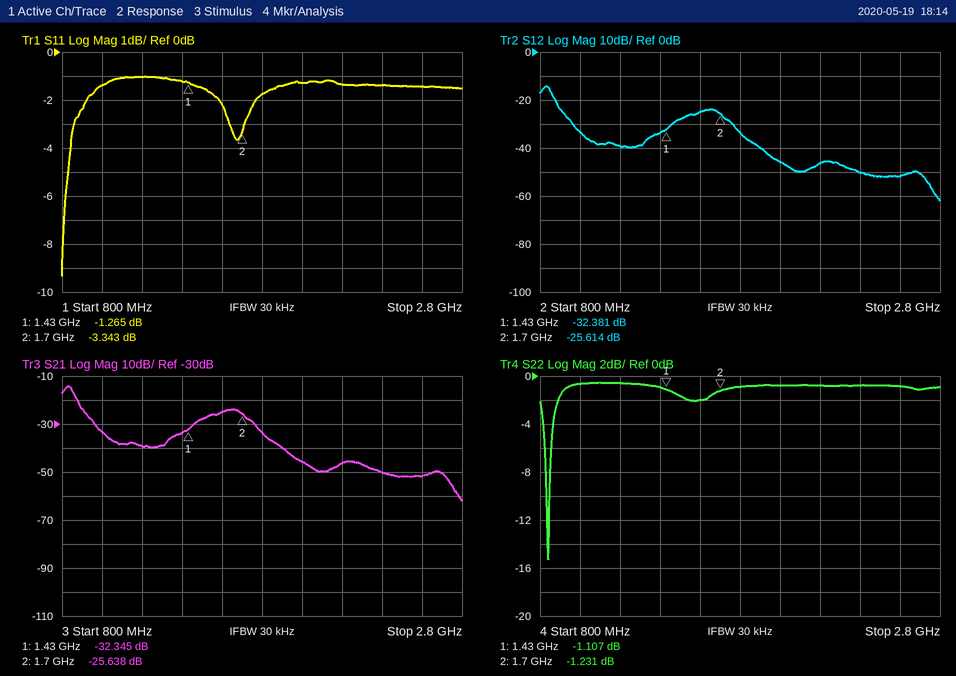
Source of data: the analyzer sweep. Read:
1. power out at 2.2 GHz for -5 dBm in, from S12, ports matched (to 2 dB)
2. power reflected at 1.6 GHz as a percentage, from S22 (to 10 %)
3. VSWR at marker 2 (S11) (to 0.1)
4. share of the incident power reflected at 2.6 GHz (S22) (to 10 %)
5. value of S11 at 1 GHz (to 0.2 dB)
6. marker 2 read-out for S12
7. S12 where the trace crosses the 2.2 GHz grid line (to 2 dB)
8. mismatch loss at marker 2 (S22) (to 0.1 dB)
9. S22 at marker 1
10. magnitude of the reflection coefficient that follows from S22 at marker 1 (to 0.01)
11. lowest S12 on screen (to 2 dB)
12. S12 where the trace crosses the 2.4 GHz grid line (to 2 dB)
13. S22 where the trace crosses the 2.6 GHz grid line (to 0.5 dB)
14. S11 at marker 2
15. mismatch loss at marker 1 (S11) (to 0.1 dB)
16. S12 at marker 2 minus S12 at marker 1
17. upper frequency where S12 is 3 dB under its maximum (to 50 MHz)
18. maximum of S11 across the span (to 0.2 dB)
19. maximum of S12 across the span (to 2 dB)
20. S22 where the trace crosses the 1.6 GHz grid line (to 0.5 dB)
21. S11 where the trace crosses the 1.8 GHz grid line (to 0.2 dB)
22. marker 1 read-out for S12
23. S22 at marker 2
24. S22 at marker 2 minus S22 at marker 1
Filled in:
-52 dBm
60 %
5.3
80 %
-1.4 dB
-25.614 dB
-46 dB
6.1 dB
-1.107 dB
0.88
-62 dB
-50 dB
-1.0 dB
-3.343 dB
6.0 dB
6.767 dB
850 MHz
-1.0 dB
-14 dB
-2.0 dB
-1.8 dB
-32.381 dB
-1.231 dB
-0.124 dB
